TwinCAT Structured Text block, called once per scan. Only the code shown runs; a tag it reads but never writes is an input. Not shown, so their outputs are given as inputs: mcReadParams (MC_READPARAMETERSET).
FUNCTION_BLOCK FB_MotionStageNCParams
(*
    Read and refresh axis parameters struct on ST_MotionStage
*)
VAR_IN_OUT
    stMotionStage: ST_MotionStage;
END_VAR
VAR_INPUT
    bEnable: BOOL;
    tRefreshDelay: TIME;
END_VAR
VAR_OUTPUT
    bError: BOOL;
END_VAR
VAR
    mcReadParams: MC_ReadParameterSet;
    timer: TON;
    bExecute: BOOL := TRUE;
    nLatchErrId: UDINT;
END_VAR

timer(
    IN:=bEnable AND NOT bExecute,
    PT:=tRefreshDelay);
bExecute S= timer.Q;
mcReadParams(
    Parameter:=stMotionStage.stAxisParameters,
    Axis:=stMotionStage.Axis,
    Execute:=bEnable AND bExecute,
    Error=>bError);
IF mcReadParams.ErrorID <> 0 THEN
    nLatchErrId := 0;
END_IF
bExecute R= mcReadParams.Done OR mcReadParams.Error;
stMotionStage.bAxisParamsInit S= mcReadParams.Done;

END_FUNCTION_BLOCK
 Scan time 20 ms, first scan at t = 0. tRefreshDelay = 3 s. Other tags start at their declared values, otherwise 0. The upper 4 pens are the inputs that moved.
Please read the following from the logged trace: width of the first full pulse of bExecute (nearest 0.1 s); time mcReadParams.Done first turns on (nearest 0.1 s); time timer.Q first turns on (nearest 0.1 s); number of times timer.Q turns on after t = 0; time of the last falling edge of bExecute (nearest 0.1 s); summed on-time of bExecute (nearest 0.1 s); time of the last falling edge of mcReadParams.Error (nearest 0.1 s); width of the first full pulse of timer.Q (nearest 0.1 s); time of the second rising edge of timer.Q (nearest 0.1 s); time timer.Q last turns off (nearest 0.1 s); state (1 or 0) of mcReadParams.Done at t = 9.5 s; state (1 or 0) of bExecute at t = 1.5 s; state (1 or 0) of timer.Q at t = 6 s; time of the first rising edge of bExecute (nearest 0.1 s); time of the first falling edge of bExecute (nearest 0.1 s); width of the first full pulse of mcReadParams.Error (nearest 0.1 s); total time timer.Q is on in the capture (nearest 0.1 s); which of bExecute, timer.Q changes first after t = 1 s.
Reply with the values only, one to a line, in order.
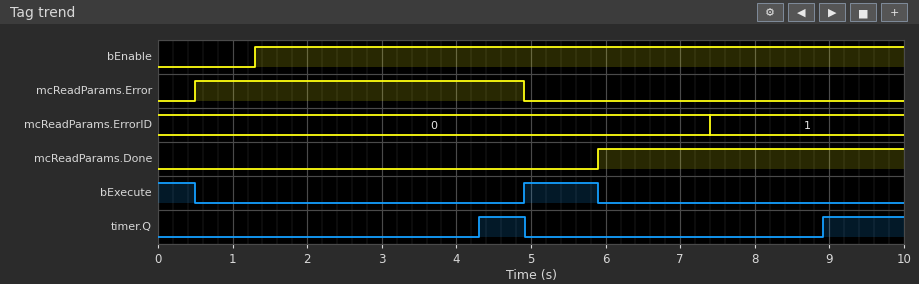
1.0 s
5.9 s
4.3 s
2
5.9 s
1.5 s
4.9 s
0.6 s
8.9 s
4.9 s
1
0
0
4.9 s
0.5 s
4.4 s
1.7 s
timer.Q
